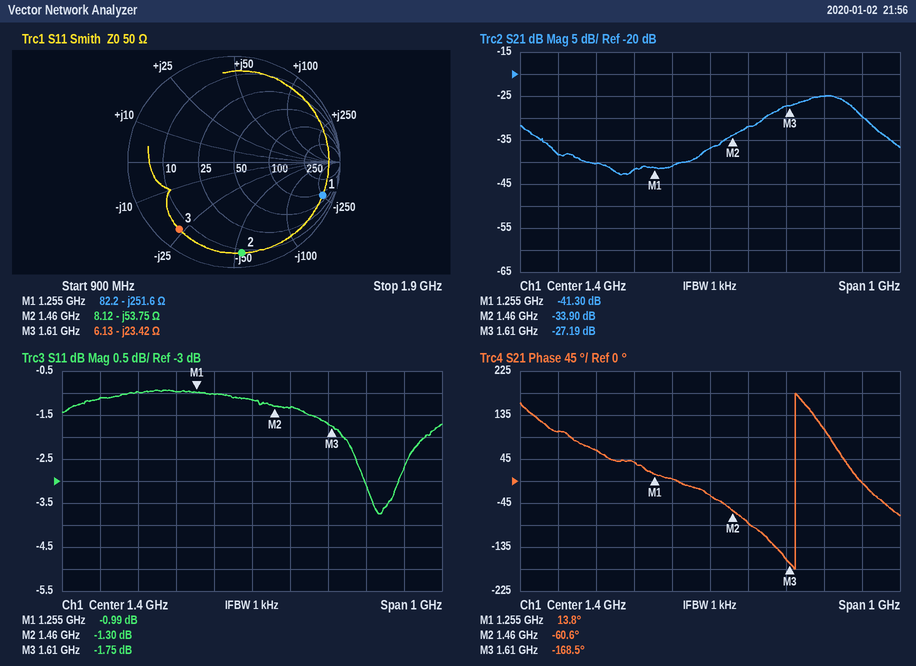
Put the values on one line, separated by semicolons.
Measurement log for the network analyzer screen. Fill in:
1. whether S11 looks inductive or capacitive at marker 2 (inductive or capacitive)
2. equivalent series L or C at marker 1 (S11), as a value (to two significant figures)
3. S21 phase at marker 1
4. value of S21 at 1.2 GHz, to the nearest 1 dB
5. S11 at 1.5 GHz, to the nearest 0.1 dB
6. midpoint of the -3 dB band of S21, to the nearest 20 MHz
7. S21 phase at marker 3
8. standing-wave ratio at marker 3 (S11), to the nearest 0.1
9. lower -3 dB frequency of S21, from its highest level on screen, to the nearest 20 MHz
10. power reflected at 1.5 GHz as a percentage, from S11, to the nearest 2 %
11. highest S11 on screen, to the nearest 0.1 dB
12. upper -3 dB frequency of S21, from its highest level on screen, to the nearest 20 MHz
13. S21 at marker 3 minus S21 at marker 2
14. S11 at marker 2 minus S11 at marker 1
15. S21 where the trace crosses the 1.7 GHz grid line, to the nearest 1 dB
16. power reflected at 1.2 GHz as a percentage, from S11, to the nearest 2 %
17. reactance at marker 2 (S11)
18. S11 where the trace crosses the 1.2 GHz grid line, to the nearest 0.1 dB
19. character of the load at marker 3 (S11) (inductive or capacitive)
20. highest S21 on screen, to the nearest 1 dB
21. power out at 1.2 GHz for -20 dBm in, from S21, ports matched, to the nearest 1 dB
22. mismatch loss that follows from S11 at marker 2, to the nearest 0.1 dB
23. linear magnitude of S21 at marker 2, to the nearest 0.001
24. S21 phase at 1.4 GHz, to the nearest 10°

capacitive; 500 fF; 13.8°; -42 dB; -1.3 dB; 1.68 GHz; -168.5°; 10.0; 1.58 GHz; 74 %; -0.9 dB; 1.78 GHz; 6.71 dB; -0.31 dB; -25 dB; 80 %; -53.75 Ω; -1.0 dB; capacitive; -25 dB; -62 dBm; 5.9 dB; 0.020; -30°
